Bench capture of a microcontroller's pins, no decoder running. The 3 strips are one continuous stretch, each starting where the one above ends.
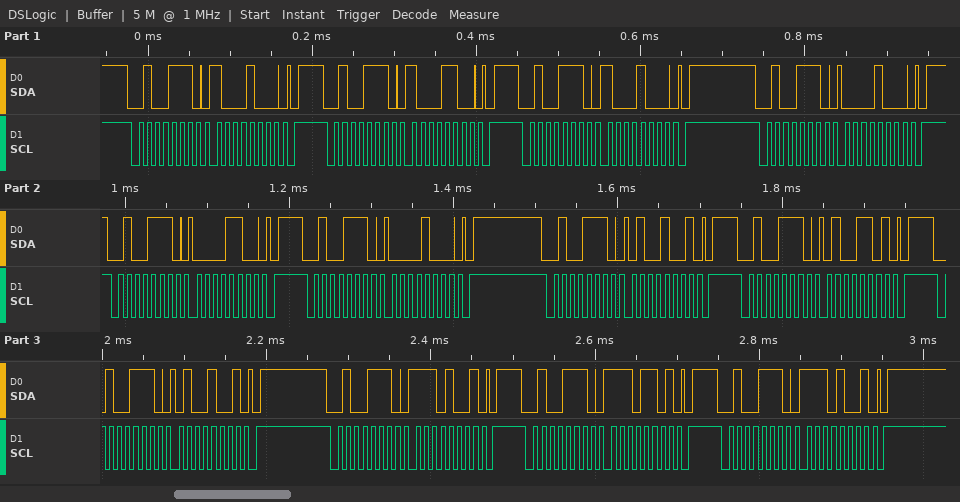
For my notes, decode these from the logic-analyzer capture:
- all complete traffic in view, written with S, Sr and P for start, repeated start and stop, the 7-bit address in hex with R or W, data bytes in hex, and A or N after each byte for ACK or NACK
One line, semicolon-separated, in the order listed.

S 27W A 88 A P S 27W A 8C A P S 27W A 88 A P S 27W A 08 A P S 27W A 0C A P S 27W A 08 A P S 27W A 49 A P S 27W A 4D A P S 27W A 49 A P S 27W A E9 A P S 27W A ED A P S 27W A E9 A P
